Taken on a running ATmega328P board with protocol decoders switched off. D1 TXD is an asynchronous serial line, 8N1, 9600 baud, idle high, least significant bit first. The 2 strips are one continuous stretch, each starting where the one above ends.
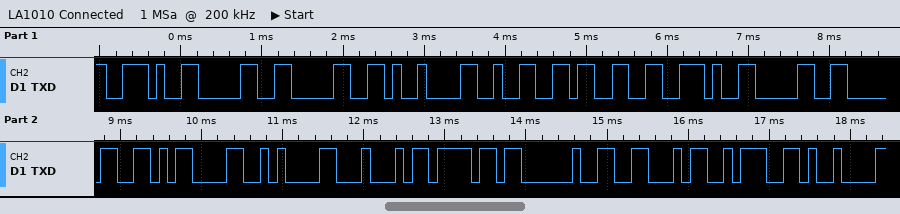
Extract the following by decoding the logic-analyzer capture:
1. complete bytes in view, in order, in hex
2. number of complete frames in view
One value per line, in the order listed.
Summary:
0x2E 0x30 0x30 0x09 0x32 0x33 0x2E 0x30 0x30 0x0D 0x0A 0x44 0x6F 0x20 0x46 0x3A 0x09
17
